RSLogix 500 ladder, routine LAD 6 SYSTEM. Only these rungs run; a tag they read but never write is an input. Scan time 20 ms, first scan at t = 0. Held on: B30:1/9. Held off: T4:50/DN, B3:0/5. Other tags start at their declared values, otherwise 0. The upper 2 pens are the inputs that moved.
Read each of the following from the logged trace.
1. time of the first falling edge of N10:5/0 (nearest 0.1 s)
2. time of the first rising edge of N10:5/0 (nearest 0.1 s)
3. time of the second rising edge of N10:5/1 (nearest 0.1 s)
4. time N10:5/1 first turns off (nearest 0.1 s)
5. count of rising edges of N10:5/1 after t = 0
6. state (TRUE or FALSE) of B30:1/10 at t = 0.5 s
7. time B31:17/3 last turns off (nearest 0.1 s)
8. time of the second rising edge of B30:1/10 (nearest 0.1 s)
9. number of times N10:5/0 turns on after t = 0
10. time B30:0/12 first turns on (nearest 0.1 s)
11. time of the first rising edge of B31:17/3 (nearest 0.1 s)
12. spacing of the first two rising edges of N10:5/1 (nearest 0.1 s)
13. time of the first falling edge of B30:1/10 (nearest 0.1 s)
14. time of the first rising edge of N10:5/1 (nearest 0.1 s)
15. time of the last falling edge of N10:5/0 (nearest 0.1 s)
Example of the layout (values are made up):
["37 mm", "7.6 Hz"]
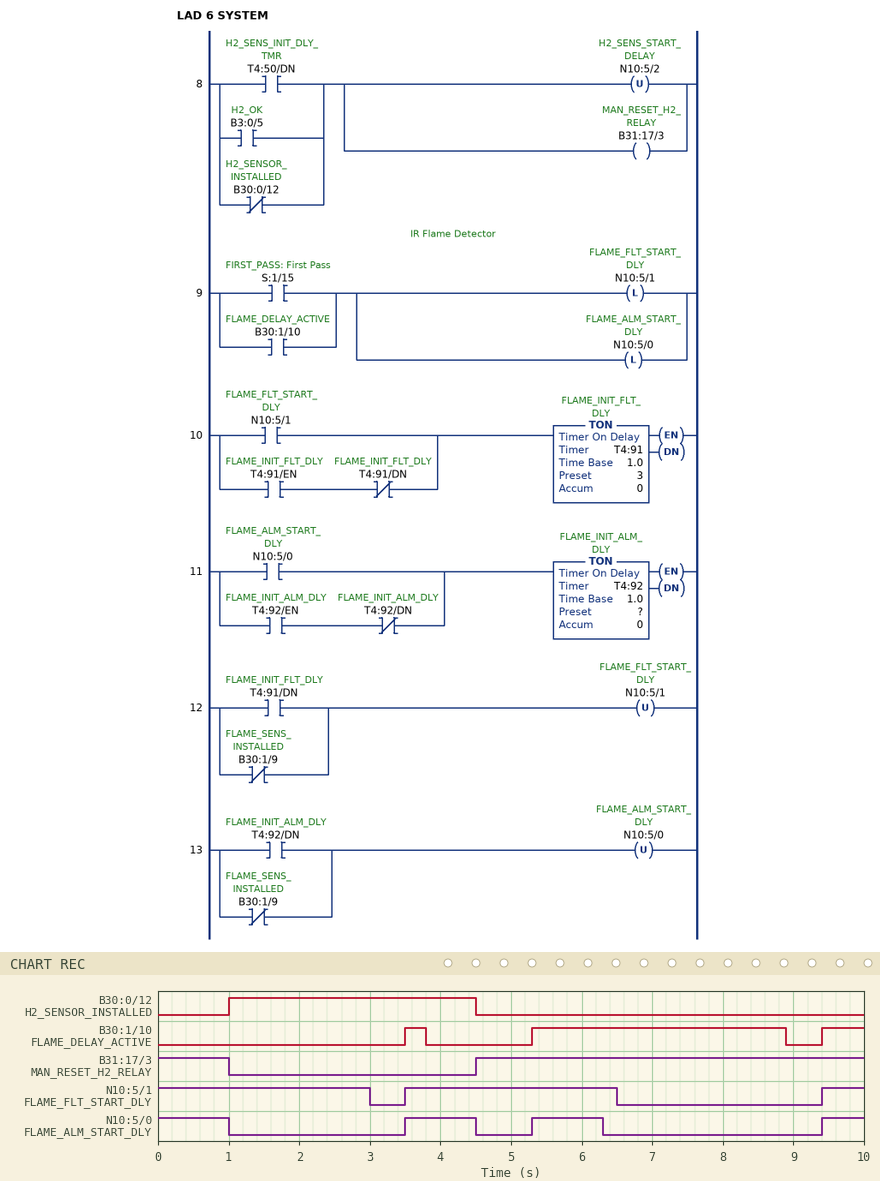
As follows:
["1.0 s", "3.5 s", "9.4 s", "3.0 s", "2", "FALSE", "1.0 s", "5.3 s", "3", "1.0 s", "4.5 s", "5.9 s", "3.8 s", "3.5 s", "6.3 s"]
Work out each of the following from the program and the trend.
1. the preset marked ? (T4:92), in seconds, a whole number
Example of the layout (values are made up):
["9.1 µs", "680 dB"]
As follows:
["1 s"]
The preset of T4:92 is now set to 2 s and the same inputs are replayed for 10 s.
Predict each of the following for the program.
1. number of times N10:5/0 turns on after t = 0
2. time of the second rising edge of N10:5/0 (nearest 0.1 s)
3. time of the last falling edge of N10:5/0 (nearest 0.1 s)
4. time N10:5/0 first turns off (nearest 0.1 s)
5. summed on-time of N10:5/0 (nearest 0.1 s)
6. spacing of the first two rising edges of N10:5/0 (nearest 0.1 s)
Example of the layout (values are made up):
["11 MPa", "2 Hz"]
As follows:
["2", "9.4 s", "5.5 s", "2.0 s", "4.6 s", "5.9 s"]
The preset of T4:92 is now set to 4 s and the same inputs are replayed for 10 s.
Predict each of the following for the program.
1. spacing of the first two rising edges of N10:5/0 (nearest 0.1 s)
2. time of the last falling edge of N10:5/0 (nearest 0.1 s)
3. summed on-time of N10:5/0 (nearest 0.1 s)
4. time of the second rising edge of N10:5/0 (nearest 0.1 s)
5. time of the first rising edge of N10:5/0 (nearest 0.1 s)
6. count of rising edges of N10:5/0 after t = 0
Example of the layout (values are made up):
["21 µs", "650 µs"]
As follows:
["4.1 s", "9.3 s", "8.6 s", "9.4 s", "5.3 s", "2"]
